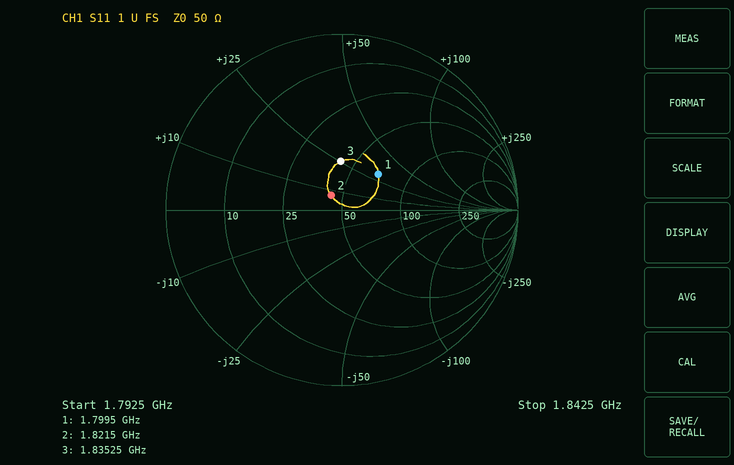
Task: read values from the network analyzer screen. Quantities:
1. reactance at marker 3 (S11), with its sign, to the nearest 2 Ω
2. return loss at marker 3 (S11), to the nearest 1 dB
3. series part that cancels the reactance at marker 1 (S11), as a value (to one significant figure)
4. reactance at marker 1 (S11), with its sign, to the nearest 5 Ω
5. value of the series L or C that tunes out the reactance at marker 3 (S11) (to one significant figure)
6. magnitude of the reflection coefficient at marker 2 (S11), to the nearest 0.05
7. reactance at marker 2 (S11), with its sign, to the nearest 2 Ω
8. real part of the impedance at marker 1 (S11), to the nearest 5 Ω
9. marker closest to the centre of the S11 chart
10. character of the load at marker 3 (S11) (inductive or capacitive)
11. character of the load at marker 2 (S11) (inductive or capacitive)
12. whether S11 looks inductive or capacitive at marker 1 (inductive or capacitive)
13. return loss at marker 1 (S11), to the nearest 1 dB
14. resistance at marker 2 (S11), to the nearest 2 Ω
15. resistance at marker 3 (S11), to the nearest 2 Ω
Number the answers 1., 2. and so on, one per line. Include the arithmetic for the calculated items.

1. +26 Ω
2. 11 dB
3. C = 1/(2π × 1.7995 GHz × 30 Ω) ≈ 3 pF
4. +30 Ω
5. C = 1/(2π × 1.83525 GHz × 26 Ω) ≈ 3 pF
6. 0.10
7. +8 Ω
8. 70 Ω
9. marker 2
10. inductive
11. inductive
12. inductive
13. 11 dB
14. 44 Ω
15. 42 Ω
